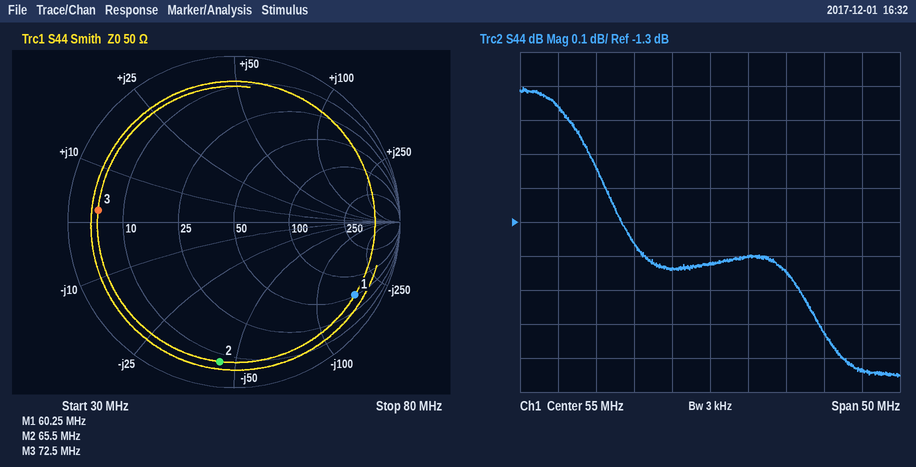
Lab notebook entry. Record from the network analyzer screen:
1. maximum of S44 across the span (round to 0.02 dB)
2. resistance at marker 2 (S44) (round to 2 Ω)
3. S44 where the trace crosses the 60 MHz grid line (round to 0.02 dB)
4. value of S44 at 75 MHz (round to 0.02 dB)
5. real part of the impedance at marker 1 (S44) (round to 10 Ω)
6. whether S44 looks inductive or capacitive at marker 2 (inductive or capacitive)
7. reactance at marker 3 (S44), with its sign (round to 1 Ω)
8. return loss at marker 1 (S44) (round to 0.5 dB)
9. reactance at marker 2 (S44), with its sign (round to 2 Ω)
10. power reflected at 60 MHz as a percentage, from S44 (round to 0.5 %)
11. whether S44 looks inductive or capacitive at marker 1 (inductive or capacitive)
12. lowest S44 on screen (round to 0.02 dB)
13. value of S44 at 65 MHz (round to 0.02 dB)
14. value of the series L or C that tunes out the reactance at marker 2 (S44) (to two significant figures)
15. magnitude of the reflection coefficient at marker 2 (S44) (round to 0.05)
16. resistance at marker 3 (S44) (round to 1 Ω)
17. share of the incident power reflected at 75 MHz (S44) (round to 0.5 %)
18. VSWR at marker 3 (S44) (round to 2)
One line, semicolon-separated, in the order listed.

-0.90 dB; 8 Ω; -1.40 dB; -1.74 dB; 50 Ω; capacitive; +2 Ω; 1.5 dB; -44 Ω; 72.5 %; capacitive; -1.76 dB; -1.44 dB; 110 nH; 0.85; 5 Ω; 67.0 %; 10
